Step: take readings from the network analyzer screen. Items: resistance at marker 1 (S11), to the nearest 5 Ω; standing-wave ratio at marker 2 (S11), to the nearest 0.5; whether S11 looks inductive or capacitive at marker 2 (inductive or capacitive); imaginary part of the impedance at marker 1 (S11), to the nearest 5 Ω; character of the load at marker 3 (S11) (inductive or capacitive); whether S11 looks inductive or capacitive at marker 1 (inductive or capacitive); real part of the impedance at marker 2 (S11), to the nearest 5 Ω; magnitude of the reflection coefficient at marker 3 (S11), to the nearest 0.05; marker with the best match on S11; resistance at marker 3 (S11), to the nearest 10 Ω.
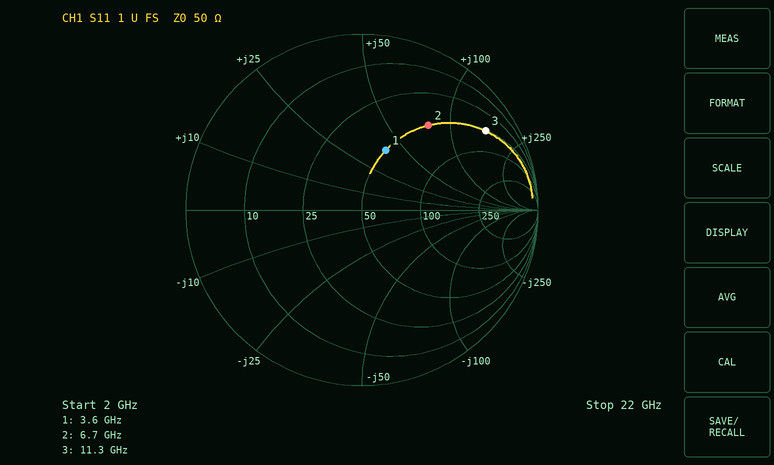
50 Ω
4.0
inductive
+40 Ω
inductive
inductive
50 Ω
0.85
marker 1
50 Ω
